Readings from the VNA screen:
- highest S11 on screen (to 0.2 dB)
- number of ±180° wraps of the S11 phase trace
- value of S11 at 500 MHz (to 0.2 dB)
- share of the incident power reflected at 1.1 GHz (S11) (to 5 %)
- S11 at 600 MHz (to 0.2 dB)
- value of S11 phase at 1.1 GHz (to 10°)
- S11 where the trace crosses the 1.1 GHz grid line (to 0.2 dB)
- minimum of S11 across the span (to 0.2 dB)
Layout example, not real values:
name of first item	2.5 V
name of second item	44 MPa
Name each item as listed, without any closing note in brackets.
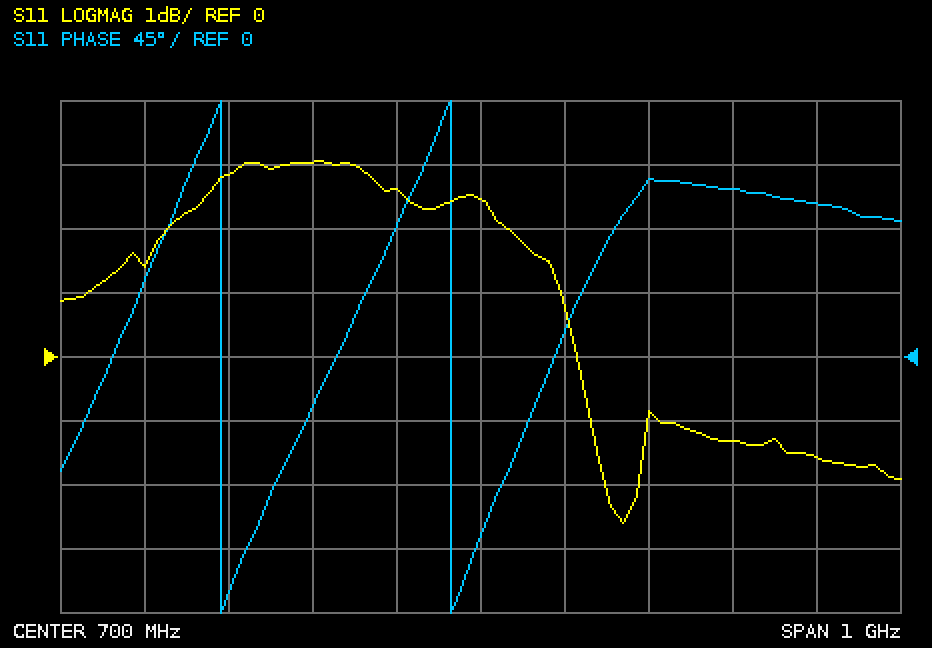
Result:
highest S11 on screen	3.0 dB
number of ±180° wraps of the S11 phase trace	2
value of S11 at 500 MHz	3.0 dB
share of the incident power reflected at 1.1 GHz (S11)	70 %
S11 at 600 MHz	2.6 dB
value of S11 phase at 1.1 GHz	110°
S11 where the trace crosses the 1.1 GHz grid line	-1.6 dB
minimum of S11 across the span	-2.6 dB
